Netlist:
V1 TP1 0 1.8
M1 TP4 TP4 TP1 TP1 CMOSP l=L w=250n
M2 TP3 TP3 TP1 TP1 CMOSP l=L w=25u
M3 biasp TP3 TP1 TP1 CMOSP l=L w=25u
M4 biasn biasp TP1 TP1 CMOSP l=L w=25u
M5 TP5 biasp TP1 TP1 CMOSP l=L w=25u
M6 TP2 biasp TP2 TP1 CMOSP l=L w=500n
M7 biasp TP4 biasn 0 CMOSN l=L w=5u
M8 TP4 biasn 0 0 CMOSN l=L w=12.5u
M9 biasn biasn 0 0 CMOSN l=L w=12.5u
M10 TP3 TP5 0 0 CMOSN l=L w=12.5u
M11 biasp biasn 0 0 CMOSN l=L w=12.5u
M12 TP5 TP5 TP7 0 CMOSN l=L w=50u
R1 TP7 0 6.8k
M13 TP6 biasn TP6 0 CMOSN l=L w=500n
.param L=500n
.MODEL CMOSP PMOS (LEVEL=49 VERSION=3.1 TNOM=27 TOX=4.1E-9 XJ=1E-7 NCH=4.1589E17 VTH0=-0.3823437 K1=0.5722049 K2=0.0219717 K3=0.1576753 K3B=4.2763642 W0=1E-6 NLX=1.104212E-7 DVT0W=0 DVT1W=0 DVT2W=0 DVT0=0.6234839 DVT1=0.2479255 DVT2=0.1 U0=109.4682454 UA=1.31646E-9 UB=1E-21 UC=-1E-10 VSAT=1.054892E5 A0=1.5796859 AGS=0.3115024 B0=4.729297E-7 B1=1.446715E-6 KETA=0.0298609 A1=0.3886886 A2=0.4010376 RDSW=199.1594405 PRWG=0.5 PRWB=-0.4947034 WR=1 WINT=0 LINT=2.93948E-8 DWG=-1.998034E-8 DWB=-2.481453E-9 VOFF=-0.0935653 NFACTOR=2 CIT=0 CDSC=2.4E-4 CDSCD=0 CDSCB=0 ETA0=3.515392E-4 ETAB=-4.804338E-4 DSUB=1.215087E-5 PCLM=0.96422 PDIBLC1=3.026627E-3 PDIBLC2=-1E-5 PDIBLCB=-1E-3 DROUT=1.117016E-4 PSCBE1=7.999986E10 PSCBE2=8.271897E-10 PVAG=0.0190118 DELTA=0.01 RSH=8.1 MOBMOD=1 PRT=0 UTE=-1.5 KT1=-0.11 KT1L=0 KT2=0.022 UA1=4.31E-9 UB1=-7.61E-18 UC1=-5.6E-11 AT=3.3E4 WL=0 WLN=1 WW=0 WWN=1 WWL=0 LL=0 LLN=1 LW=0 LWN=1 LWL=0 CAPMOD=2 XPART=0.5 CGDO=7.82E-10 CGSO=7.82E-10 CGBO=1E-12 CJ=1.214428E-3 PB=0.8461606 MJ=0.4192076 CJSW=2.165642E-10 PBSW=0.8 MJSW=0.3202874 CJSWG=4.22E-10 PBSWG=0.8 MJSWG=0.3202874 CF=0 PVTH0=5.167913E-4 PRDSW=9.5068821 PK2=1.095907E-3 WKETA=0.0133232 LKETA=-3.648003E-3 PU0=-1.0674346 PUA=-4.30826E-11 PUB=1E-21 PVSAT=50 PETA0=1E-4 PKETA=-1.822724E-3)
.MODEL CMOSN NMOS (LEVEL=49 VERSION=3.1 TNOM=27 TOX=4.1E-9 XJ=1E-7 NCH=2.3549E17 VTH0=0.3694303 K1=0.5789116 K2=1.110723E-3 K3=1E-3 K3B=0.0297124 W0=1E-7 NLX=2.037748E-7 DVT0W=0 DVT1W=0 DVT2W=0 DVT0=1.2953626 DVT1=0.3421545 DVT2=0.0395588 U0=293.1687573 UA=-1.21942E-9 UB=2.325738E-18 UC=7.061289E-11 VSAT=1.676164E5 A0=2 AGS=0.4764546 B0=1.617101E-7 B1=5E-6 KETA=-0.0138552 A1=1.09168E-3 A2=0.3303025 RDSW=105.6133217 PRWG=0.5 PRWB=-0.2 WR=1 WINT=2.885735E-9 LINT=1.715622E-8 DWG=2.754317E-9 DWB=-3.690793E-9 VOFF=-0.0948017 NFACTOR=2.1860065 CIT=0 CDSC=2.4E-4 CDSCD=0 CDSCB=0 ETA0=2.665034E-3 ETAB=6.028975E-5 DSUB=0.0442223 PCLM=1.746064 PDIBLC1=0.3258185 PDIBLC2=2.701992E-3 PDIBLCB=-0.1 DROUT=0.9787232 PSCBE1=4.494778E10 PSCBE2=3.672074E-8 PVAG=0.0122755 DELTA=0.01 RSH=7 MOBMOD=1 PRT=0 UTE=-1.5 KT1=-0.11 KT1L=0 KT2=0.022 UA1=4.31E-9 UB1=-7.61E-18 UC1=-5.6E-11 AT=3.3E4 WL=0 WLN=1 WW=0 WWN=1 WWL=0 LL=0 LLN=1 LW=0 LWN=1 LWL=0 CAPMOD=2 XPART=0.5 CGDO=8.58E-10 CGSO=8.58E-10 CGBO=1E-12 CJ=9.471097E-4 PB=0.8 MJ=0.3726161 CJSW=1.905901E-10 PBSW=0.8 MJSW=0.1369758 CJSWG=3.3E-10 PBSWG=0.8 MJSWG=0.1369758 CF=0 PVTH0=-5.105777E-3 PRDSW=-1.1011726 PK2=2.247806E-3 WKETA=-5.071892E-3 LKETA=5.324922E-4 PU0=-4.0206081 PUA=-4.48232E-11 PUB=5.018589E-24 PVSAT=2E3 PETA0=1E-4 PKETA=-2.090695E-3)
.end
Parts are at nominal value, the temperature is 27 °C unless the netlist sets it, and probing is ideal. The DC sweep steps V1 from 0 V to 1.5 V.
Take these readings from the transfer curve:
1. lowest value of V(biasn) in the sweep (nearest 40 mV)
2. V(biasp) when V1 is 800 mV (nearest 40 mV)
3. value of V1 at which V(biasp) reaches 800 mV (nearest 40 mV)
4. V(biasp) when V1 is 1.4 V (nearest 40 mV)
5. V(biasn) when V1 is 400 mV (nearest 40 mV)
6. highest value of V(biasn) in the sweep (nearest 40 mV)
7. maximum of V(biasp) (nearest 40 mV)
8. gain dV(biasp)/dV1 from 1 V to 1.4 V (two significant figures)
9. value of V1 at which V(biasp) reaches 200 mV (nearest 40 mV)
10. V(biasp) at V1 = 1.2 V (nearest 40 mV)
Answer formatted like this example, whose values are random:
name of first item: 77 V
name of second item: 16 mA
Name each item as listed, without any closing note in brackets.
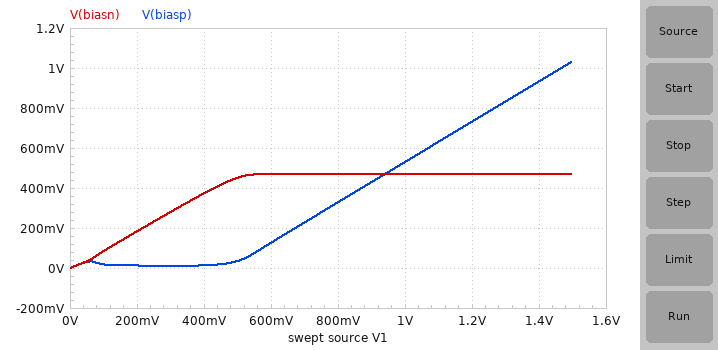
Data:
lowest value of V(biasn) in the sweep: 0 V
V(biasp) when V1 is 800 mV: 320 mV
value of V1 at which V(biasp) reaches 800 mV: 1.28 V
V(biasp) when V1 is 1.4 V: 920 mV
V(biasn) when V1 is 400 mV: 360 mV
highest value of V(biasn) in the sweep: 480 mV
maximum of V(biasp): 1.04 V
gain dV(biasp)/dV1 from 1 V to 1.4 V: 1.0 V/V
value of V1 at which V(biasp) reaches 200 mV: 680 mV
V(biasp) at V1 = 1.2 V: 720 mV
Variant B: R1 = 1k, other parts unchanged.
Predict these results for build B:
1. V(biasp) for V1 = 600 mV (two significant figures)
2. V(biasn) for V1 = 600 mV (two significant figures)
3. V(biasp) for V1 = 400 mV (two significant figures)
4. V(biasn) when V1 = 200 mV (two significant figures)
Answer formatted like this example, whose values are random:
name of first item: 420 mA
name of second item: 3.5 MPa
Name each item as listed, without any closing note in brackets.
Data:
V(biasp) for V1 = 600 mV: 35 mV
V(biasn) for V1 = 600 mV: 530 mV
V(biasp) for V1 = 400 mV: 11 mV
V(biasn) when V1 = 200 mV: 180 mV
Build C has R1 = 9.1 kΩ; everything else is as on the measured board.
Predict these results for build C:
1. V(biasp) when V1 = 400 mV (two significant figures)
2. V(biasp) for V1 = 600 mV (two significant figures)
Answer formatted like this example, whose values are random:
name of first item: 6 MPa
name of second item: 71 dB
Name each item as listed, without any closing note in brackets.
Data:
V(biasp) when V1 = 400 mV: 14 mV
V(biasp) for V1 = 600 mV: 140 mV
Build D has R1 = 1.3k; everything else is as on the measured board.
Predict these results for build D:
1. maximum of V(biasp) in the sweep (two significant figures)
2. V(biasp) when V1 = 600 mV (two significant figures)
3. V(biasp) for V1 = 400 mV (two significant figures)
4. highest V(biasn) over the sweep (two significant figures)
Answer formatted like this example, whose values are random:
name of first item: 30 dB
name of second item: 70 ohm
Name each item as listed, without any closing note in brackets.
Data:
maximum of V(biasp) in the sweep: 910 mV
V(biasp) when V1 = 600 mV: 41 mV
V(biasp) for V1 = 400 mV: 11 mV
highest V(biasn) over the sweep: 570 mV
